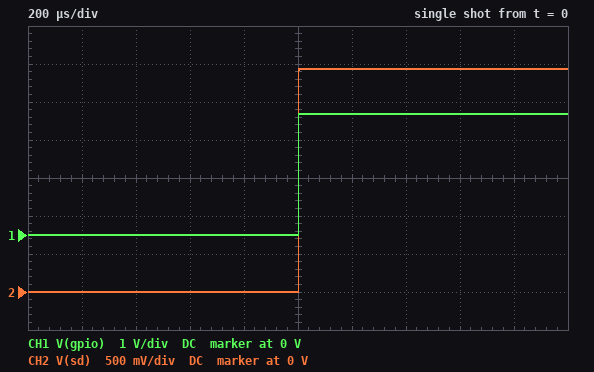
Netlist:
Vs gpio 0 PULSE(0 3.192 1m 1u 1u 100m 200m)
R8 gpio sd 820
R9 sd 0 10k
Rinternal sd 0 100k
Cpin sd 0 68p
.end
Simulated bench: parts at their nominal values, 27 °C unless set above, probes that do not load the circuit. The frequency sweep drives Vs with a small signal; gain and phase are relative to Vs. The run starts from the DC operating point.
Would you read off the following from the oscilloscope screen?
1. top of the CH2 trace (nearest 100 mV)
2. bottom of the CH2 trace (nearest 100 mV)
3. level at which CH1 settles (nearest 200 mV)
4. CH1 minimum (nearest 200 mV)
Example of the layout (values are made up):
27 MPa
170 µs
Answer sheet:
2.9 V
0 V
3.2 V
0 V
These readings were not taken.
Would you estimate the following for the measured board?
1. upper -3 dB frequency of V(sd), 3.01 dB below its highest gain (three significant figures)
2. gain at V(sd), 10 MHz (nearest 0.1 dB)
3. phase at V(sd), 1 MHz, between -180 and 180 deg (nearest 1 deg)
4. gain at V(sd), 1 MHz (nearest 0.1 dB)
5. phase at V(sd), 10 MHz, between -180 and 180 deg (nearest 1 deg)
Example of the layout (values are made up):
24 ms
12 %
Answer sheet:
3.11 MHz
-11.3 dB
-18 deg
-1.2 dB
-73 deg
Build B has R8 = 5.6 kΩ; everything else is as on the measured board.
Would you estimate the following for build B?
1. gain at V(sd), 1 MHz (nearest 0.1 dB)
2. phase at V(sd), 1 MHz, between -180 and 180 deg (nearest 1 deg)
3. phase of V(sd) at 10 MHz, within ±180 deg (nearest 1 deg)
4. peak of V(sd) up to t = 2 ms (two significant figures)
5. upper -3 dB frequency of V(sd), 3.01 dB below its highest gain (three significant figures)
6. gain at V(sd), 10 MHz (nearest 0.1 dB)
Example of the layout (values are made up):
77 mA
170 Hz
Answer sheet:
-9.2 dB
-56 deg
-86 deg
2.0 V
675 kHz
-27.6 dB
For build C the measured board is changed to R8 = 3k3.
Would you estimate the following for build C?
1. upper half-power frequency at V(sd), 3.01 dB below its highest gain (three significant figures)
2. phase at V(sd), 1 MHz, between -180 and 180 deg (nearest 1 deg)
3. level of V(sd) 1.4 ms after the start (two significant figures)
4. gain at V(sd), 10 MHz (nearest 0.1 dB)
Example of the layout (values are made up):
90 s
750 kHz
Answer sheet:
967 kHz
-46 deg
2.3 V
-23.0 dB
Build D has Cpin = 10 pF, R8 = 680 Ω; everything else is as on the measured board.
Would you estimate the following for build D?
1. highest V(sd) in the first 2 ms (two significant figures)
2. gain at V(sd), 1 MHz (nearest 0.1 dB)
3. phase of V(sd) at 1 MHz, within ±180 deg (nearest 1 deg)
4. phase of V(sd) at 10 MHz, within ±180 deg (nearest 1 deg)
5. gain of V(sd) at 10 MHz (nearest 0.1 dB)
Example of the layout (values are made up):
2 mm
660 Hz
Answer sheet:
3.0 V
-0.6 dB
-2 deg
-22 deg
-1.3 dB
